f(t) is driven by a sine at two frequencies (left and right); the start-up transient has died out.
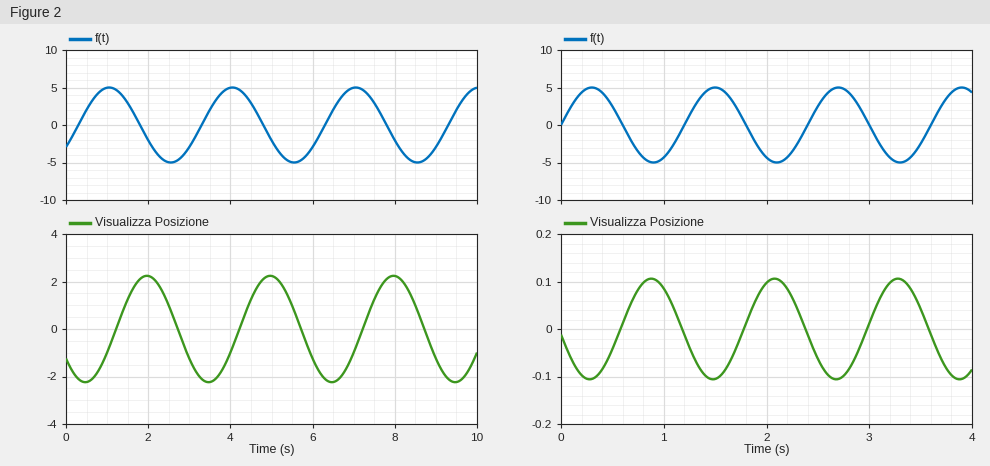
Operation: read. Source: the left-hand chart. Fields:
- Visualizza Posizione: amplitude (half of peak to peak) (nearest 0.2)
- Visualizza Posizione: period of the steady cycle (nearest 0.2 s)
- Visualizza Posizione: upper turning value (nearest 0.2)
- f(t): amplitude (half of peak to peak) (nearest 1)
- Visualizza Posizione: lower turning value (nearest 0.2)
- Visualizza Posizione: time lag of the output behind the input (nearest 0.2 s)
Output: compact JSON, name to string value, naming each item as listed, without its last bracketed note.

{"Visualizza Posizione: amplitude (half of peak to peak)": "2.2", "Visualizza Posizione: period of the steady cycle": "3.0 s", "Visualizza Posizione: upper turning value": "2.2", "f(t): amplitude (half of peak to peak)": "5", "Visualizza Posizione: lower turning value": "-2.2", "Visualizza Posizione: time lag of the output behind the input": "1.0 s"}
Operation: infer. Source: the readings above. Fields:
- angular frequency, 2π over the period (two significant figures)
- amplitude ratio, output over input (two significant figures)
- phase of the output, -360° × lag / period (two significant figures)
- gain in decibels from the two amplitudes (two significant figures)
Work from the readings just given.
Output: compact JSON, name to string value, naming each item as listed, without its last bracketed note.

{"angular frequency, 2π over the period": "2.1 rad/s", "amplitude ratio, output over input": "0.44", "phase of the output, -360° × lag / period": "-120°", "gain in decibels from the two amplitudes": "-7.1 dB"}
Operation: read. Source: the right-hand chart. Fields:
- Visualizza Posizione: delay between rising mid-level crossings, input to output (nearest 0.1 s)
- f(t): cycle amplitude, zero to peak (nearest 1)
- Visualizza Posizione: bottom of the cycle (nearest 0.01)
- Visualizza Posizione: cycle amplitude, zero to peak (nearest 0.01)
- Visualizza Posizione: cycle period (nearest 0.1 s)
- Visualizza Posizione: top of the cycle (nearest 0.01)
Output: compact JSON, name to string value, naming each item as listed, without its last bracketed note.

{"Visualizza Posizione: delay between rising mid-level crossings, input to output": "0.6 s", "f(t): cycle amplitude, zero to peak": "5", "Visualizza Posizione: bottom of the cycle": "-0.11", "Visualizza Posizione: cycle amplitude, zero to peak": "0.11", "Visualizza Posizione: cycle period": "1.2 s", "Visualizza Posizione: top of the cycle": "0.11"}
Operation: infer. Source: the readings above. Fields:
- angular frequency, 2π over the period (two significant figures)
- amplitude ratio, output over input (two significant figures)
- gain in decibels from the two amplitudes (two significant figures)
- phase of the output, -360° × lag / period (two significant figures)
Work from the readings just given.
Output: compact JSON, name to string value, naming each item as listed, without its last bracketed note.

{"angular frequency, 2π over the period": "5.2 rad/s", "amplitude ratio, output over input": "0.022", "gain in decibels from the two amplitudes": "-33 dB", "phase of the output, -360° × lag / period": "-180°"}
